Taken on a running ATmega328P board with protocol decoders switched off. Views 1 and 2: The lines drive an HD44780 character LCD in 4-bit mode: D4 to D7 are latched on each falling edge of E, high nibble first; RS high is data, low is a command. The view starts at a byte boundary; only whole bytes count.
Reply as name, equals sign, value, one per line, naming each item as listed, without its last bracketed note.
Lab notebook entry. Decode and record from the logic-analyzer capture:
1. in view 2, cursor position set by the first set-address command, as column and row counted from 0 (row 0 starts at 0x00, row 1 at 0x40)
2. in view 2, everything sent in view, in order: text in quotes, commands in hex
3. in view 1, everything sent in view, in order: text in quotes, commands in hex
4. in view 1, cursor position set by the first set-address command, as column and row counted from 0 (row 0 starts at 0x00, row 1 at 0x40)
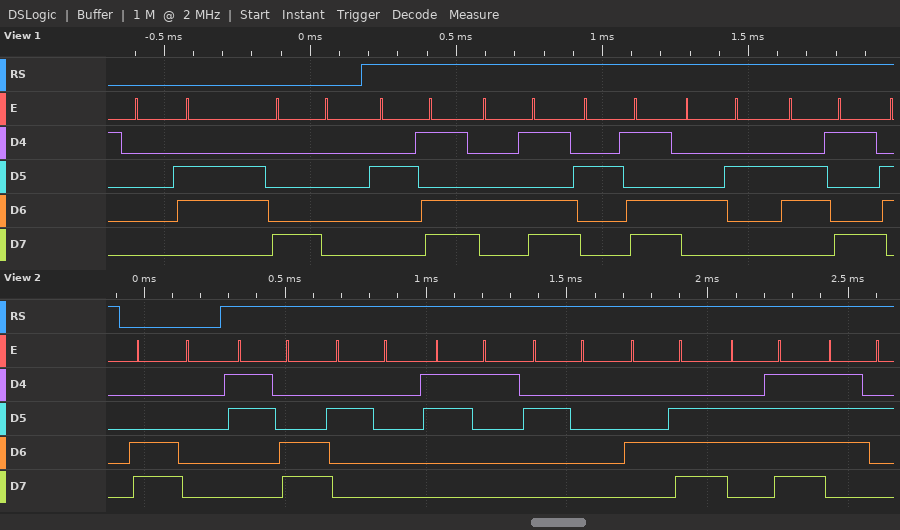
in view 2, cursor position set by the first set-address command, as column and row counted from 0 = column 0, row 1
in view 2, everything sent in view, in order: text in quotes, commands in hex = 0xC0 "< 1 Nor"
in view 1, everything sent in view, in order: text in quotes, commands in hex = 0x06 0x80 "-M-Bi"
in view 1, cursor position set by the first set-address command, as column and row counted from 0 = column 0, row 0
